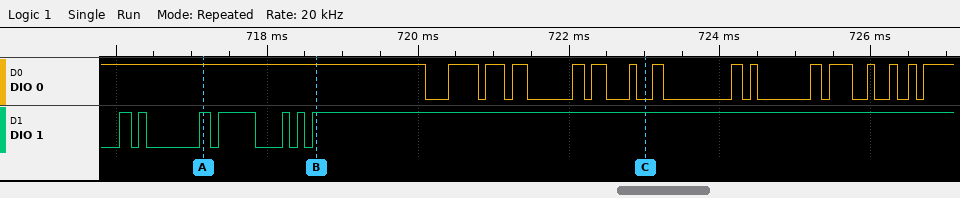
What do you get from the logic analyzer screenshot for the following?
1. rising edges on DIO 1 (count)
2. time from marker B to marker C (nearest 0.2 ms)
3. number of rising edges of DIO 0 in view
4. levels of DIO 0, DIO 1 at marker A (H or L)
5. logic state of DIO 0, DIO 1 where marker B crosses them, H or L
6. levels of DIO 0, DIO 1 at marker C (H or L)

7
4.4 ms
15
DIO 0=H, DIO 1=H
DIO 0=H, DIO 1=H
DIO 0=L, DIO 1=H
